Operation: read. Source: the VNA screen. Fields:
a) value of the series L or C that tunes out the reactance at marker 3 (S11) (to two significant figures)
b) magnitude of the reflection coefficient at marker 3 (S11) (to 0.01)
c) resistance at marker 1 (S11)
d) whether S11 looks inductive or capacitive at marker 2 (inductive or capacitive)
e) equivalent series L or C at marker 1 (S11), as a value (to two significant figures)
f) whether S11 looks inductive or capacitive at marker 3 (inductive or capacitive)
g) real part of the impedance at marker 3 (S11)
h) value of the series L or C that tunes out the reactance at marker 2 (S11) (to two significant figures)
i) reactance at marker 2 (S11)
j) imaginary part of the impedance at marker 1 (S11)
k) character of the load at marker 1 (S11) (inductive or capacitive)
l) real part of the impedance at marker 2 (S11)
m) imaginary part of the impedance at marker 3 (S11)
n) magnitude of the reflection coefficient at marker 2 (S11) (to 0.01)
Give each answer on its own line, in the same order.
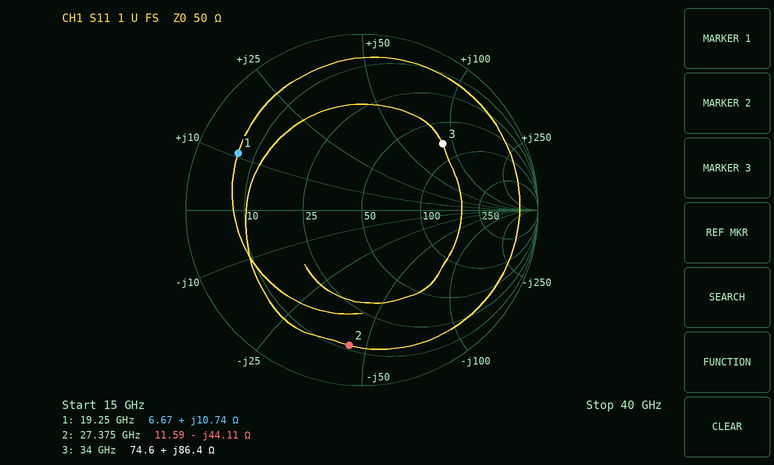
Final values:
54 fF
0.59
6.67 Ω
capacitive
89 pH
inductive
74.6 Ω
260 pH
-44.11 Ω
+10.74 Ω
inductive
11.59 Ω
+86.4 Ω
0.77
